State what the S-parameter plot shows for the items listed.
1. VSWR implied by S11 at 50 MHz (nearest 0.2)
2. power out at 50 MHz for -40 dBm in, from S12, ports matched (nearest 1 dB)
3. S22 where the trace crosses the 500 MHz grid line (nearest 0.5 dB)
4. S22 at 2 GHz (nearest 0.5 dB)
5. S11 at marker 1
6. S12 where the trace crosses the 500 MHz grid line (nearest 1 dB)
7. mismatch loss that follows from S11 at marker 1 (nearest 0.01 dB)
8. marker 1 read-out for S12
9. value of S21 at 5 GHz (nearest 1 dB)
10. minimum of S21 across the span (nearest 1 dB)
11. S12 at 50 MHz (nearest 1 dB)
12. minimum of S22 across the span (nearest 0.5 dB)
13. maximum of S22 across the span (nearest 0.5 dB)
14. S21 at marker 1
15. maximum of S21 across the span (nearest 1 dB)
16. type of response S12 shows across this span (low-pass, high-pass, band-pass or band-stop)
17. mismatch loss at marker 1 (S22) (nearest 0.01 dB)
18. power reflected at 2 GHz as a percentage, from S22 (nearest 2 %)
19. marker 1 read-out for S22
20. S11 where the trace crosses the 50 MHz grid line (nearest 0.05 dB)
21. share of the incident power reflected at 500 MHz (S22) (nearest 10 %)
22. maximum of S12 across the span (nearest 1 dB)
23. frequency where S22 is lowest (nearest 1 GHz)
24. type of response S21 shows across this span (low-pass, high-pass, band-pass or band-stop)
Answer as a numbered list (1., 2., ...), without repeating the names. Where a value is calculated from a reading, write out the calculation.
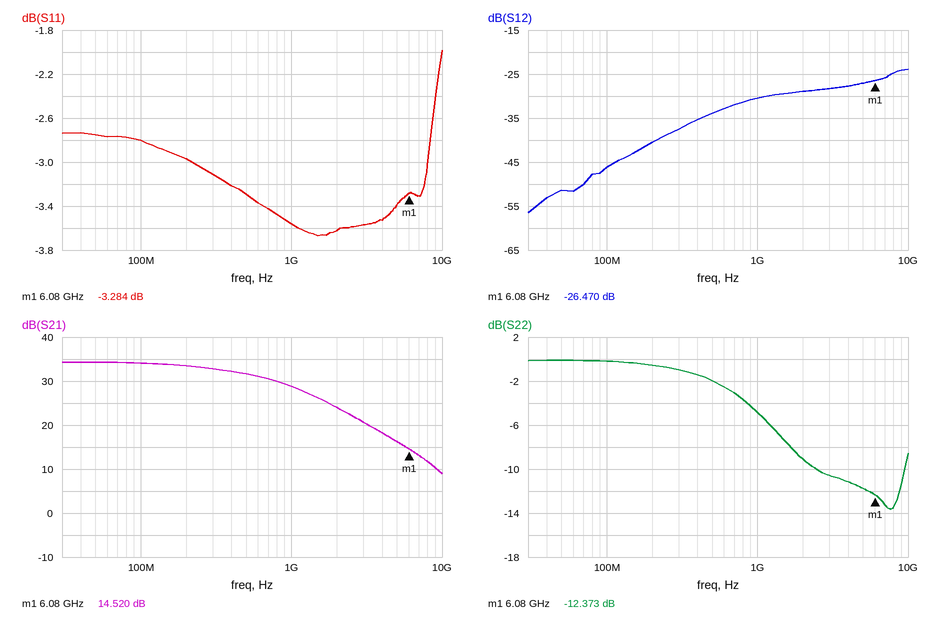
1. |Γ| = 10^(-2.75/20) = 0.7286; VSWR = (1 + 0.7286)/(1 − 0.7286) ≈ 6.4
2. -40 dBm + (-51 dB) = -91 dBm
3. -2.0 dB
4. -9.0 dB
5. -3.284 dB
6. -34 dB
7. −10 log10(1 − 10^(-3.284/10)) ≈ 2.75 dB
8. -26.470 dB
9. 16 dB
10. 9 dB
11. -51 dB
12. -13.5 dB
13. 0.0 dB
14. 14.520 dB
15. 34 dB
16. high-pass
17. −10 log10(1 − 10^(-12.373/10)) ≈ 0.26 dB
18. 10^(-9/10) ≈ 12.6 %, so 12 % to the nearest 2 %
19. -12.373 dB
20. -2.75 dB
21. 10^(-2/10) ≈ 63.1 %, so 60 % to the nearest 10 %
22. -24 dB
23. 8 GHz
24. low-pass
